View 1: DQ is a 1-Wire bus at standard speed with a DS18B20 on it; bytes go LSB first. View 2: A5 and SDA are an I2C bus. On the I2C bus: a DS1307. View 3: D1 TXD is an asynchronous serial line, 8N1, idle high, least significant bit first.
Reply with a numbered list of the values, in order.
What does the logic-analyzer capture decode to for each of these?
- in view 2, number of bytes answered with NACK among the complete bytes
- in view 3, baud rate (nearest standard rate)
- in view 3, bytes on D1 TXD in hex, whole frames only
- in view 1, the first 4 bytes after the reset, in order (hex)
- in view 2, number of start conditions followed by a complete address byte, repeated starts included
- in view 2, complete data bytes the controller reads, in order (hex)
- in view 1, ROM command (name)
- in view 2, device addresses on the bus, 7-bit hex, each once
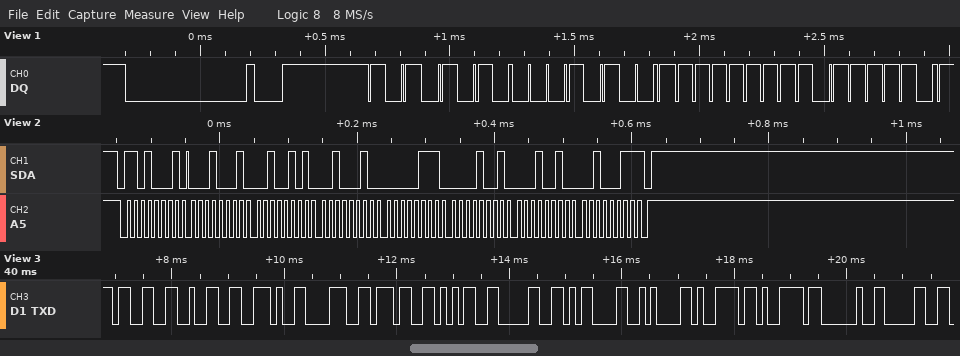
1. 1
2. 9600 baud
3. 33 32 2E 38 37 35 30 0D 0A 79 79 20 30
4. 55 28 FF 7D
5. 1
6. 11 25 22 07 09 12 23
7. Match ROM
8. 0x68
